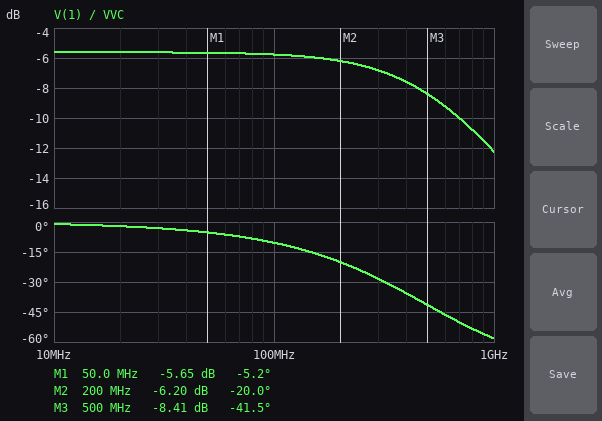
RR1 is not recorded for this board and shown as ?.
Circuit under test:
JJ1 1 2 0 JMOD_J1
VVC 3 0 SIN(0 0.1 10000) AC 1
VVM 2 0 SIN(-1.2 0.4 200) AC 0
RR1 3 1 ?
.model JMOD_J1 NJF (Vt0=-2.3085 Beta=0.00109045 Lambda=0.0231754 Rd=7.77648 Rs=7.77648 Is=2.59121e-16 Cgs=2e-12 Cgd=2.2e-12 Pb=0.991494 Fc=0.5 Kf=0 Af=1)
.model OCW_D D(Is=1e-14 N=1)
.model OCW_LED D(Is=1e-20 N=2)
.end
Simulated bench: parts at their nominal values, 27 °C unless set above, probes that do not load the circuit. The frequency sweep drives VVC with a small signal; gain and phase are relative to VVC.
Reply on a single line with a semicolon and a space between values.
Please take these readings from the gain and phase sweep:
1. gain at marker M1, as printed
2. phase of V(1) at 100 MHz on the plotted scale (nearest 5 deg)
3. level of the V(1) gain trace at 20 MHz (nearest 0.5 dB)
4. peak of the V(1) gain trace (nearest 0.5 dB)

-5.65 dB; -10 deg; -5.5 dB; -5.5 dB
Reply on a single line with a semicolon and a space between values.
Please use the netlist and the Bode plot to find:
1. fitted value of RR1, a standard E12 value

390 Ω
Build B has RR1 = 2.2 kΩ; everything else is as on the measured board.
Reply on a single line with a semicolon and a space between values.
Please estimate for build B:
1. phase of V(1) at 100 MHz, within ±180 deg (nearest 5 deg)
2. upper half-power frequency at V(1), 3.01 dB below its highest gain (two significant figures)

-20 deg; 300 MHz
